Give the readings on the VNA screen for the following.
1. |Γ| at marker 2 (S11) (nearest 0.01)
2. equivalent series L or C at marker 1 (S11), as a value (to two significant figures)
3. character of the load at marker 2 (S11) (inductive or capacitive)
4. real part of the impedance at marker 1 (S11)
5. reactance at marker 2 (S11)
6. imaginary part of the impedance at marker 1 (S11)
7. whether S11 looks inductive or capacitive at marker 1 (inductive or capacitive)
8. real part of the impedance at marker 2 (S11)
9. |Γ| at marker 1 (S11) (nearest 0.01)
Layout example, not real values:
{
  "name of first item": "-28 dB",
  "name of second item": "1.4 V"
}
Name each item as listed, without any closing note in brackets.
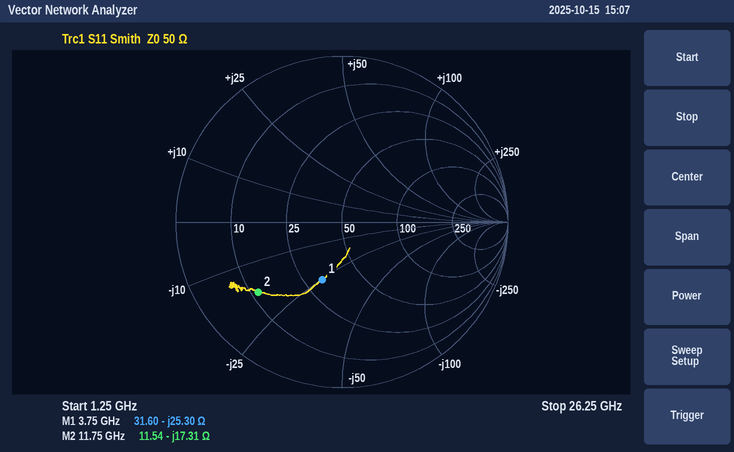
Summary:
{
  "|Γ| at marker 2 (S11)": "0.66",
  "equivalent series L or C at marker 1 (S11), as a value": "1.7 pF",
  "character of the load at marker 2 (S11)": "capacitive",
  "real part of the impedance at marker 1": "31.60 Ω",
  "reactance at marker 2": "-17.31 Ω",
  "imaginary part of the impedance at marker 1": "-25.30 Ω",
  "whether S11 looks inductive or capacitive at marker 1": "capacitive",
  "real part of the impedance at marker 2": "11.54 Ω",
  "|Γ| at marker 1 (S11)": "0.37"
}
